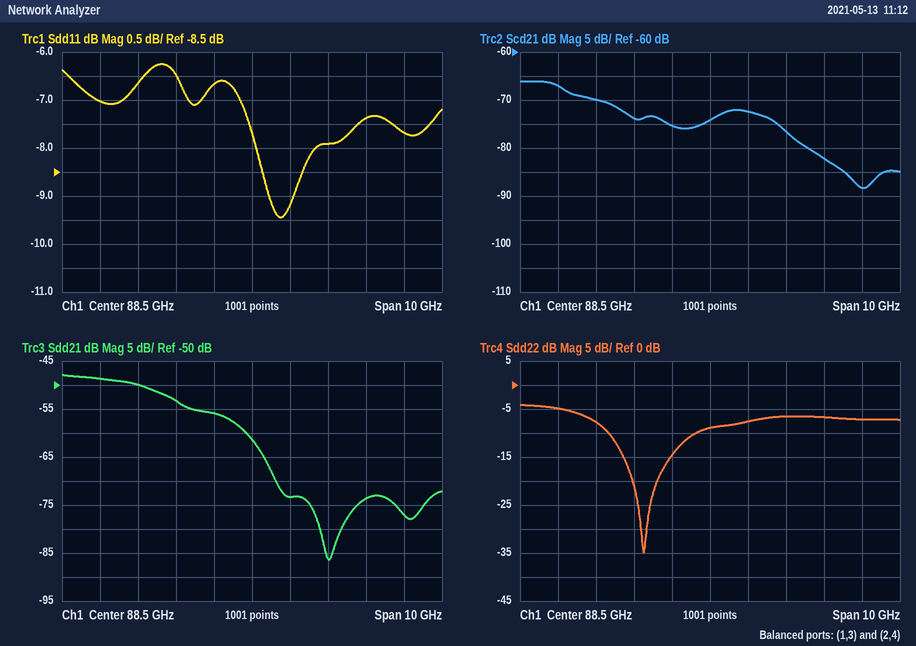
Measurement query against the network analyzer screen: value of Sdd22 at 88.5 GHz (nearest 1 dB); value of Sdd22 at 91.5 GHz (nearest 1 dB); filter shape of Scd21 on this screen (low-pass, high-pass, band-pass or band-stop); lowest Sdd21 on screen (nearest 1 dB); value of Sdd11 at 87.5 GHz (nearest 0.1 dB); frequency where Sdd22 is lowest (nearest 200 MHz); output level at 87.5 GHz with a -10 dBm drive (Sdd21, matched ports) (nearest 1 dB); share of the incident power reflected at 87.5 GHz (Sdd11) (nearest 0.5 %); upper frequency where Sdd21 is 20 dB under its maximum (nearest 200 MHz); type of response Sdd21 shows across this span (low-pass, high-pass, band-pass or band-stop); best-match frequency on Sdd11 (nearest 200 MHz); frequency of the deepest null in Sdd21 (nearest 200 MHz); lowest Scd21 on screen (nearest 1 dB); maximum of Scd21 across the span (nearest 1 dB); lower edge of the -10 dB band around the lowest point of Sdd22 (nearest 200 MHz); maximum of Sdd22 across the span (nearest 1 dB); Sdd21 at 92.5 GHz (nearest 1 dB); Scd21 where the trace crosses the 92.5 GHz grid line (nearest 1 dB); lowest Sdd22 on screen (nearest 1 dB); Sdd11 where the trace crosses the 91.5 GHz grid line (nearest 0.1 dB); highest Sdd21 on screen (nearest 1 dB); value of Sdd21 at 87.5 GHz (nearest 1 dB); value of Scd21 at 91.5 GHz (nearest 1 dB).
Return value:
-9 dB
-7 dB
low-pass
-86 dB
-6.7 dB
86.8 GHz
-66 dBm
21.5 %
89.0 GHz
low-pass
89.2 GHz
90.6 GHz
-88 dB
-66 dB
85.8 GHz
-4 dB
-77 dB
-88 dB
-35 dB
-7.4 dB
-48 dB
-56 dB
-82 dB
